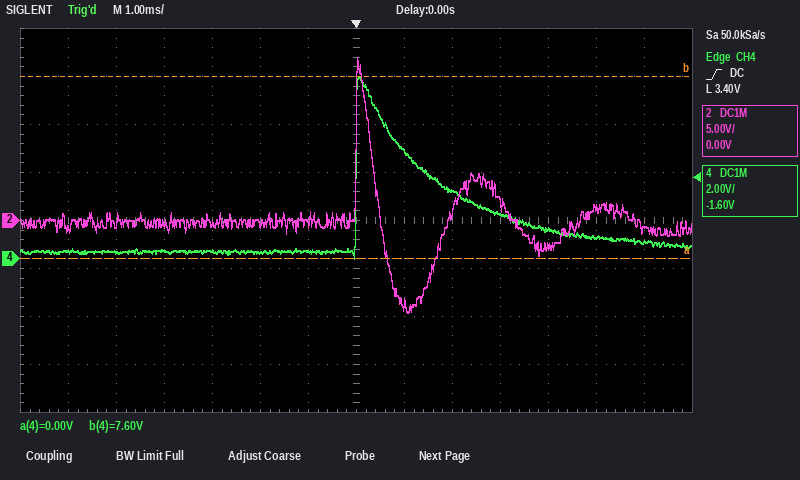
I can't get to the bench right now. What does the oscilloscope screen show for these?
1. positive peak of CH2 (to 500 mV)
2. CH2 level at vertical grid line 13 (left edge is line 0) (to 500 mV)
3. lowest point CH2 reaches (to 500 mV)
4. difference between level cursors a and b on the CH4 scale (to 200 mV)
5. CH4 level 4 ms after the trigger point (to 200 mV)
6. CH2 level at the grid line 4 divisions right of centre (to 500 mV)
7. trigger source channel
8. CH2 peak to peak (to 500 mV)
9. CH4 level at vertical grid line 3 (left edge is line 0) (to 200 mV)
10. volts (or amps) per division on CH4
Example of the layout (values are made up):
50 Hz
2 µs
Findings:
17.0 V
-1.0 V
-9.5 V
7.6 V
1.2 V
-2.5 V
CH4
26.5 V
400 mV
2 V
